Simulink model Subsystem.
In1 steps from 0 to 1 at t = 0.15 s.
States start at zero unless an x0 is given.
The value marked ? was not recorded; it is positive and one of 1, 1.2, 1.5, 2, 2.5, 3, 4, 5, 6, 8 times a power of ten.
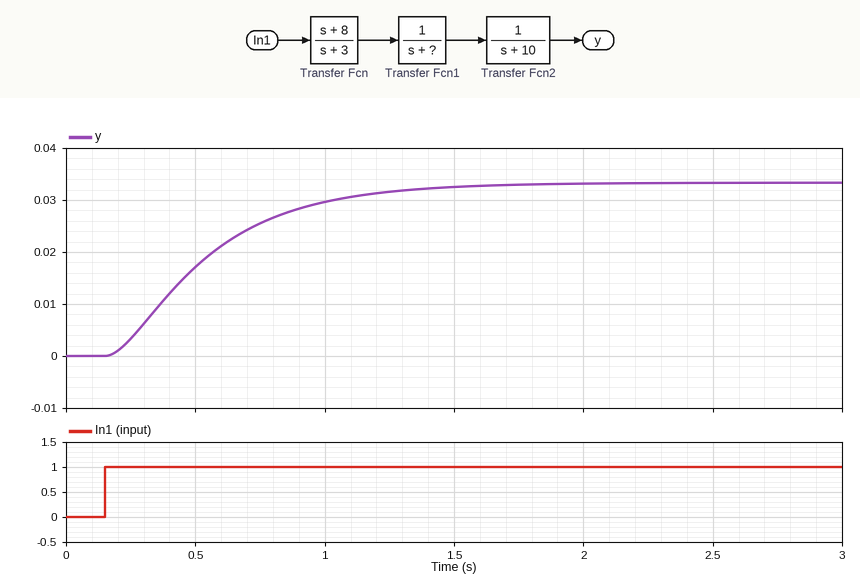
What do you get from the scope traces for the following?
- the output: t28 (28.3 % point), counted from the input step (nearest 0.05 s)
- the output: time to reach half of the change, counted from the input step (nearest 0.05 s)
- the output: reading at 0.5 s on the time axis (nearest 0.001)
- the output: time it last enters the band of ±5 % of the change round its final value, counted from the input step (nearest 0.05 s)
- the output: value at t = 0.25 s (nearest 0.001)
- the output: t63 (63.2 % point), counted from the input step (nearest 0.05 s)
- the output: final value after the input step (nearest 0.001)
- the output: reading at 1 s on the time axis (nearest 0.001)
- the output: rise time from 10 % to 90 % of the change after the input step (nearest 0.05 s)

0.20 s
0.35 s
0.017
1.10 s
0.003
0.45 s
0.033
0.030
0.80 s
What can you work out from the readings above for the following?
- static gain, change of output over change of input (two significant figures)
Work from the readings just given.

0.033
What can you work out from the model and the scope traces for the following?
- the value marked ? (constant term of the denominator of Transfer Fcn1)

8
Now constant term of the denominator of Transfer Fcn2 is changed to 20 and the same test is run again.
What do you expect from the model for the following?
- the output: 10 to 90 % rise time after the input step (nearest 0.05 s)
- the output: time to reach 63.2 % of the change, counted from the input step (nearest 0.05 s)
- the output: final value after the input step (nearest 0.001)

0.75 s
0.40 s
0.017
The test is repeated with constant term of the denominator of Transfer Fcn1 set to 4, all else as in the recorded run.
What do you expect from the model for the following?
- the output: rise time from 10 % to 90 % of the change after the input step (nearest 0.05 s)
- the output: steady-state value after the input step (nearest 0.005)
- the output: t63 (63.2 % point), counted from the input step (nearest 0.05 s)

0.95 s
0.065
0.60 s
